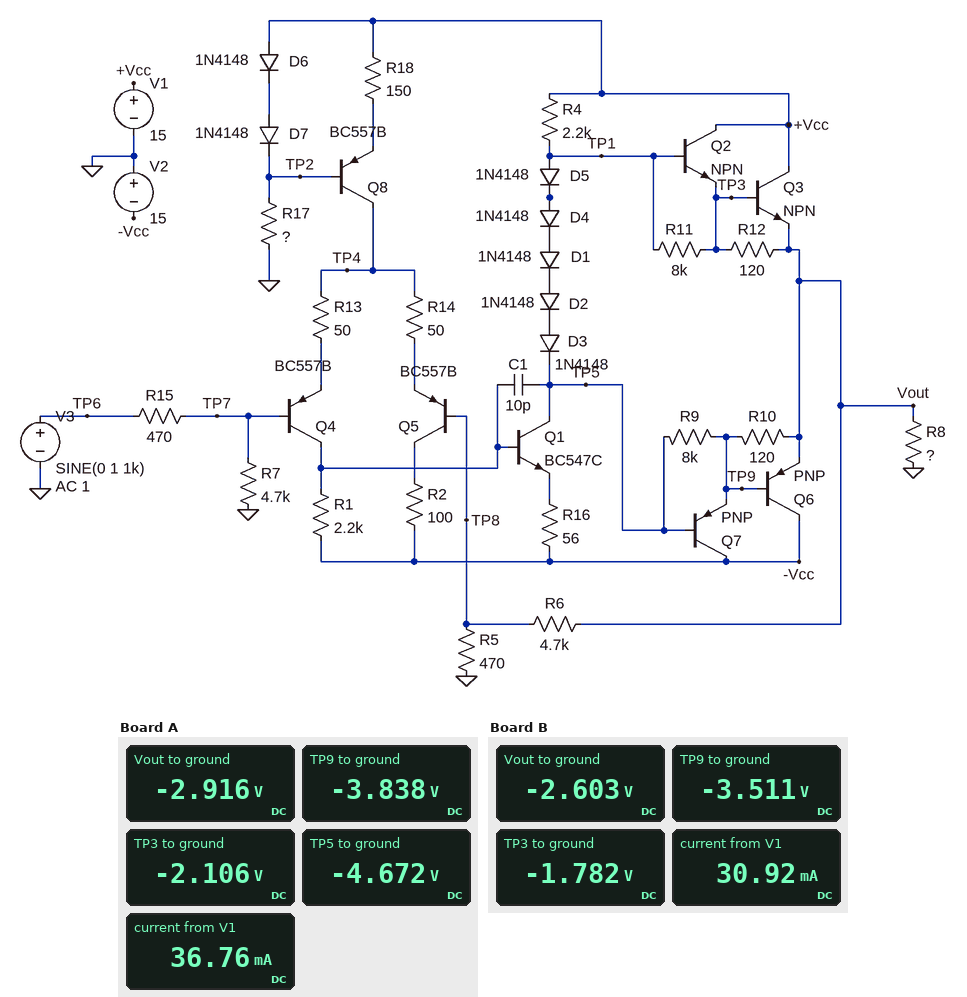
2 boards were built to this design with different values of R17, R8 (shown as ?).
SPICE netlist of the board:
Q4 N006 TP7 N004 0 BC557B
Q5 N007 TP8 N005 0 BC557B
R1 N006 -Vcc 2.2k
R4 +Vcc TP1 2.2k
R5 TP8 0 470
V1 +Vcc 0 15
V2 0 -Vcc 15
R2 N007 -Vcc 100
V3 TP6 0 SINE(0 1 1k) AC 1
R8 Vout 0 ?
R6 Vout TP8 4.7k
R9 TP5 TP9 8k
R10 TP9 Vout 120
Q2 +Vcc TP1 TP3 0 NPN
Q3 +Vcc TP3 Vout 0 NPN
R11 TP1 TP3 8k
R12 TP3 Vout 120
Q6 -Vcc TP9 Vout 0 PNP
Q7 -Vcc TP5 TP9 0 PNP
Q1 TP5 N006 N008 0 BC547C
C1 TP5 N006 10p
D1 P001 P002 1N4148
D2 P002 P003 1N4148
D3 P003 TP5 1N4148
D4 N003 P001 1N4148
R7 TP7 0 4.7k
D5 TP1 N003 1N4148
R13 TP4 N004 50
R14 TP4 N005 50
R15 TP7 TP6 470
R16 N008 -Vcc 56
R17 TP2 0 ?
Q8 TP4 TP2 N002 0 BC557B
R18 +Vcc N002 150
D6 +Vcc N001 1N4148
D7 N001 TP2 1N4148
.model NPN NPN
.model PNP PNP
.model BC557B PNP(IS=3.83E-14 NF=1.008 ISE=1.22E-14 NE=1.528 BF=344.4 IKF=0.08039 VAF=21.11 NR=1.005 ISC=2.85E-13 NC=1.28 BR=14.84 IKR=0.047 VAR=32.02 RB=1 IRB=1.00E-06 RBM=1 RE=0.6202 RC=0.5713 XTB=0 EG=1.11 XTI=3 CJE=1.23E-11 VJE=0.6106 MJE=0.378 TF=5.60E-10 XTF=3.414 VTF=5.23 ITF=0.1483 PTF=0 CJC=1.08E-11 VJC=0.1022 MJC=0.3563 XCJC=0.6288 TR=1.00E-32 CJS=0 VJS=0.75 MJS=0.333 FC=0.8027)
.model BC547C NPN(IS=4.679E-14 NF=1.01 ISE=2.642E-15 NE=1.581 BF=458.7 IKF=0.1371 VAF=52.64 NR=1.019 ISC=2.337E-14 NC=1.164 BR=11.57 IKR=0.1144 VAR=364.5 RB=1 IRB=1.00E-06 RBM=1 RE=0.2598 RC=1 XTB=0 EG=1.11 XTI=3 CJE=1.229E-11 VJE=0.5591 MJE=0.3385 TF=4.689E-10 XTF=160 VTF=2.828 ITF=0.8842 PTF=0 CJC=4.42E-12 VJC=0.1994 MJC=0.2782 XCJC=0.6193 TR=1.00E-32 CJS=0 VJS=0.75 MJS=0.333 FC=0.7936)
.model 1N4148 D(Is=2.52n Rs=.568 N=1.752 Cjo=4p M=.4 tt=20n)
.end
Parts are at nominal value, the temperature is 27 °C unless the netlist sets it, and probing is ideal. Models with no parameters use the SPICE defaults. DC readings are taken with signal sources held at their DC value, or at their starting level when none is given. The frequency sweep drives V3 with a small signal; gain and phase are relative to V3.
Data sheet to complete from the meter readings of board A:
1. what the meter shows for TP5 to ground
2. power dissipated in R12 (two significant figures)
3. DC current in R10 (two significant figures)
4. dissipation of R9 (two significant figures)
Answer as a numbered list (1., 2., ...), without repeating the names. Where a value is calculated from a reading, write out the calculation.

1. -4.672 V
2. (-2.106 V - (-2.916 V))^2 / 120 Ω = 5.5 mW
3. (-2.916 V - (-3.838 V)) / 120 Ω = 7.7 mA
4. (-3.838 V - (-4.672 V))^2 / 8 kΩ = 87 µW
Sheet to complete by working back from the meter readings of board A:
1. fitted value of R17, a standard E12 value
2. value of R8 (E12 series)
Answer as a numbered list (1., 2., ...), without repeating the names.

1. 1 kΩ
2. 10 Ω
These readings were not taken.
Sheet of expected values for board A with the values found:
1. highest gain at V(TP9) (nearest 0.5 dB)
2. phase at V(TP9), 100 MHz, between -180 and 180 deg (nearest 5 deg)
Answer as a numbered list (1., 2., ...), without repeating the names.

1. 20.0 dB
2. 125 deg
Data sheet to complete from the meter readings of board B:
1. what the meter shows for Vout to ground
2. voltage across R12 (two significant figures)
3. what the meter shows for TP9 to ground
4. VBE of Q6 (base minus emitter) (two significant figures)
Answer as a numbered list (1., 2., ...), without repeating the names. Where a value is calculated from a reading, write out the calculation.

1. -2.603 V
2. -1.782 V - (-2.603 V) = 820 mV
3. -3.511 V
4. -3.511 V - (-2.603 V) = -910 mV
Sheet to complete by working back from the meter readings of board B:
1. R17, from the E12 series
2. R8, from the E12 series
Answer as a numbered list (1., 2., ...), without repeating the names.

1. 2.2 kΩ
2. 15 Ω
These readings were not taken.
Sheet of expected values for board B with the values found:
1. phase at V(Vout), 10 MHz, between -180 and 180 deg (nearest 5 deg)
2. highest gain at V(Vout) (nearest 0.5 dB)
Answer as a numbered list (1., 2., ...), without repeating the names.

1. -95 deg
2. 20.0 dB
